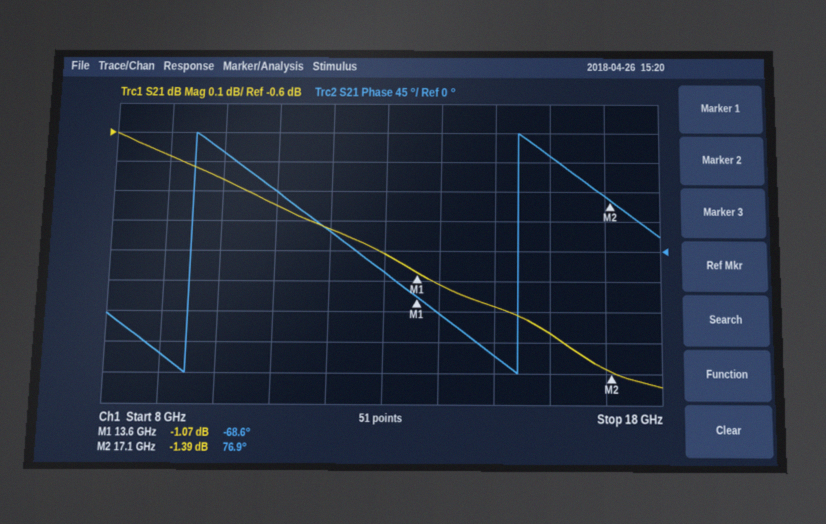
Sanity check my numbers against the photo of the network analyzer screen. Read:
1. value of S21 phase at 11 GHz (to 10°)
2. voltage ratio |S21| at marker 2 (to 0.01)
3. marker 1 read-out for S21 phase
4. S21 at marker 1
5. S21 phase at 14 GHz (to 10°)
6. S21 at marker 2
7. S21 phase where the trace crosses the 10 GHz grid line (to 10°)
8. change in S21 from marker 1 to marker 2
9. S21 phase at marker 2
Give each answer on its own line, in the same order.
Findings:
90°
0.85
-68.6°
-1.07 dB
-90°
-1.39 dB
150°
-0.32 dB
76.9°
